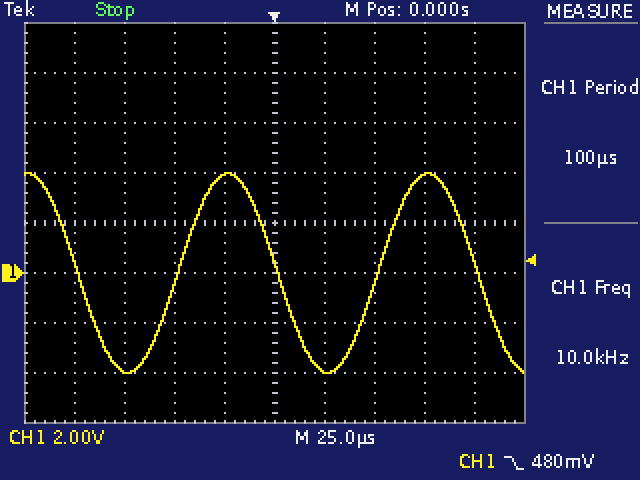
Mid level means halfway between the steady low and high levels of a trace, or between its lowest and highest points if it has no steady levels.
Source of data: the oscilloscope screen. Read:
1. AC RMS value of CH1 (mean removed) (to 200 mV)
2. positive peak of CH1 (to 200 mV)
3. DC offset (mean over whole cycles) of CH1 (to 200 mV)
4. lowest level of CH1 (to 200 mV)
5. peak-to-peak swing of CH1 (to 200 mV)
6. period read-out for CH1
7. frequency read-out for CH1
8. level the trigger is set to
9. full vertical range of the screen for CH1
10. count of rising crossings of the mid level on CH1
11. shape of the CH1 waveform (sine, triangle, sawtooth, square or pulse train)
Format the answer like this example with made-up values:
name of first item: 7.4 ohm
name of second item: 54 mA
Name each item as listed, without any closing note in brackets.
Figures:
AC RMS value of CH1 (mean removed): 2.8 V
positive peak of CH1: 4.0 V
DC offset (mean over whole cycles) of CH1: 0.0 V
lowest level of CH1: -4.0 V
peak-to-peak swing of CH1: 8.0 V
period read-out for CH1: 100 µs
frequency read-out for CH1: 10.0 kHz
level the trigger is set to: 480 mV
full vertical range of the screen for CH1: 16 V
count of rising crossings of the mid level on CH1: 2
shape of the CH1 waveform: sine
